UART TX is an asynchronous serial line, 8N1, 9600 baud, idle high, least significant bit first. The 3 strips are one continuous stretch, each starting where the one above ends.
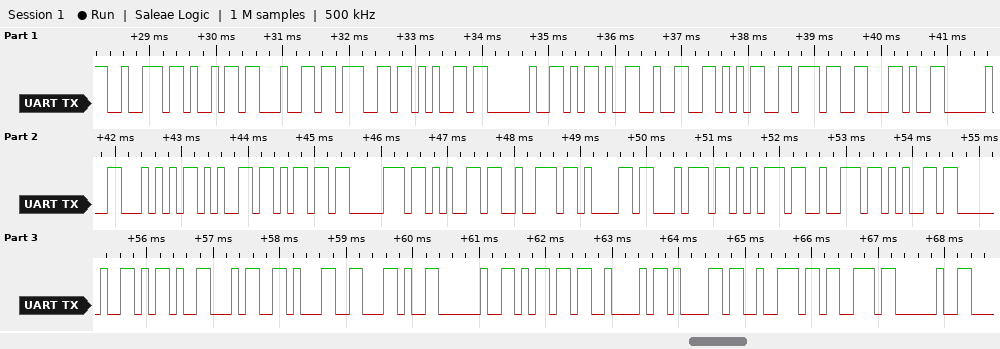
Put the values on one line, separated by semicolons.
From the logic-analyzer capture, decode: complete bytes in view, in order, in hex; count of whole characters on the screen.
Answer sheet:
0x72 0x69 0x64 0x67 0x65 0x20 0x2D 0x32 0x35 0x37 0x2C 0x20 0x54 0x65 0x6D 0x70 0x65 0x72 0x61 0x74 0x75 0x72 0x65 0x20 0x2D 0x34 0x31 0x2C 0x20 0x6D 0x42 0x61 0x72 0x73 0x20; 35
